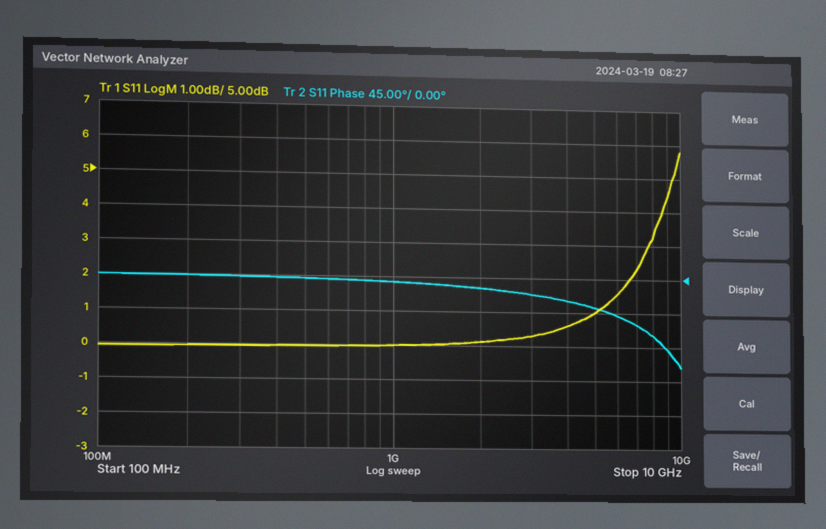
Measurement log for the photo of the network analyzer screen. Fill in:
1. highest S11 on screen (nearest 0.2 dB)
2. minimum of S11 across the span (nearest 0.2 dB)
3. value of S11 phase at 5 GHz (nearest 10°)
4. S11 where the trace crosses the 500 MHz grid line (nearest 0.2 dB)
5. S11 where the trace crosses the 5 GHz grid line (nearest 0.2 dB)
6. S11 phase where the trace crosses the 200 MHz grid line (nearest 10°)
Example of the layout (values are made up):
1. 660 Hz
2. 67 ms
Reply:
1. 5.8 dB
2. 0.0 dB
3. -40°
4. 0.0 dB
5. 1.0 dB
6. 0°
